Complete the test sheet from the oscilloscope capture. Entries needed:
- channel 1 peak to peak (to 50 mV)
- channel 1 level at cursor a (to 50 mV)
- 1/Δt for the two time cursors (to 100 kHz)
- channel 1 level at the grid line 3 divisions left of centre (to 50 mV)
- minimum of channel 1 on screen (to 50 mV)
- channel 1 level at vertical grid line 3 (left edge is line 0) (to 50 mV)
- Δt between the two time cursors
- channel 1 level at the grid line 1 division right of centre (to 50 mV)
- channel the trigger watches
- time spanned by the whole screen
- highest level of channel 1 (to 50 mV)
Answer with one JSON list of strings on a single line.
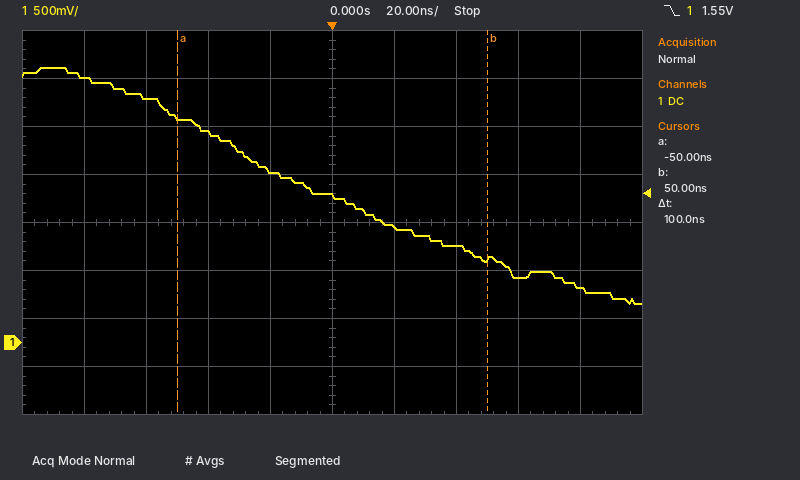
["2.45 V", "2.35 V", "10.0 MHz", "2.55 V", "400 mV", "2.20 V", "100 ns", "1.20 V", "channel 1", "200 ns", "2.85 V"]
